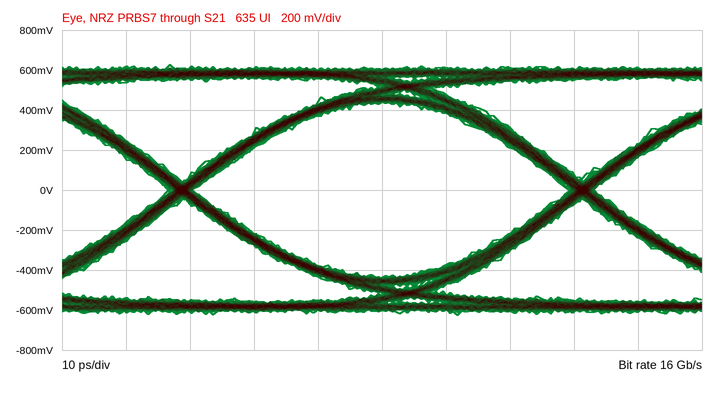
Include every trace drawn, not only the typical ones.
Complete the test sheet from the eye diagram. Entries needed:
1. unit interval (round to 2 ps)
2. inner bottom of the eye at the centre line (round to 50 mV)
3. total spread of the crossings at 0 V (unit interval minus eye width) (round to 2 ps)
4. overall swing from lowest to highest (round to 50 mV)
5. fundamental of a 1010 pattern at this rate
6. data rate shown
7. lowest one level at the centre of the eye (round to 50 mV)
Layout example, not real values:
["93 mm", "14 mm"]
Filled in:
["62 ps", "-450 mV", "4 ps", "1.25 V", "8 GHz", "16 Gb/s", "450 mV"]
